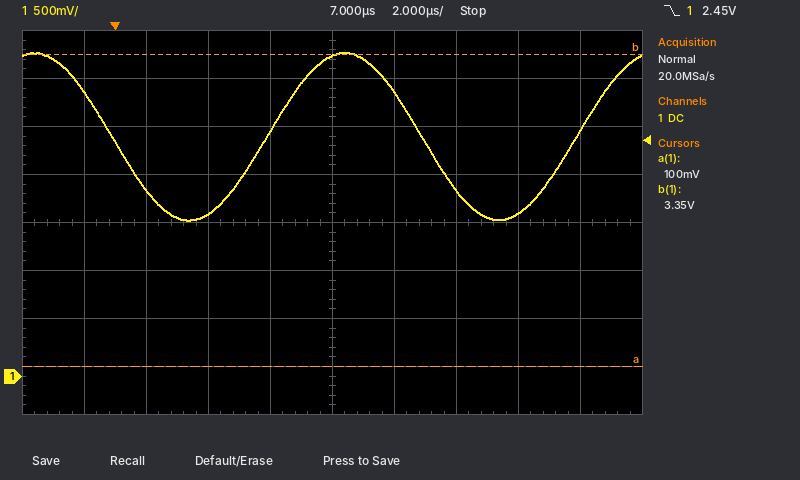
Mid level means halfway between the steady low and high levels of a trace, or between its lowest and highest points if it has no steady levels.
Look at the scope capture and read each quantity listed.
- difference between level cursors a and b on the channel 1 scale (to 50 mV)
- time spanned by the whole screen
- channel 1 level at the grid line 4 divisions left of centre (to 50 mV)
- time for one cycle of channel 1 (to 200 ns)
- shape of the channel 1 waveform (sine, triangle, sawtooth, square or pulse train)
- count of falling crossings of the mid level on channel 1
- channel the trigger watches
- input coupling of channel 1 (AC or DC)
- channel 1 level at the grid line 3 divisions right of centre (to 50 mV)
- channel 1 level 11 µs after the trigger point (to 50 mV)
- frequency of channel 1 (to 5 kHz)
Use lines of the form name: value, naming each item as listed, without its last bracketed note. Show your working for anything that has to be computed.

difference between level cursors a and b on the channel 1 scale: 3.25 V
time spanned by the whole screen: 20 µs
channel 1 level at the grid line 4 divisions left of centre: 2.95 V
time for one cycle of channel 1: 10.0 µs
shape of the channel 1 waveform: sine
count of falling crossings of the mid level on channel 1: 2
channel the trigger watches: channel 1
input coupling of channel 1: DC
channel 1 level at the grid line 3 divisions right of centre: 1.70 V
channel 1 level 11 µs after the trigger point: 1.95 V
frequency of channel 1: 1 / 10.0 µs ≈ 100 kHz
